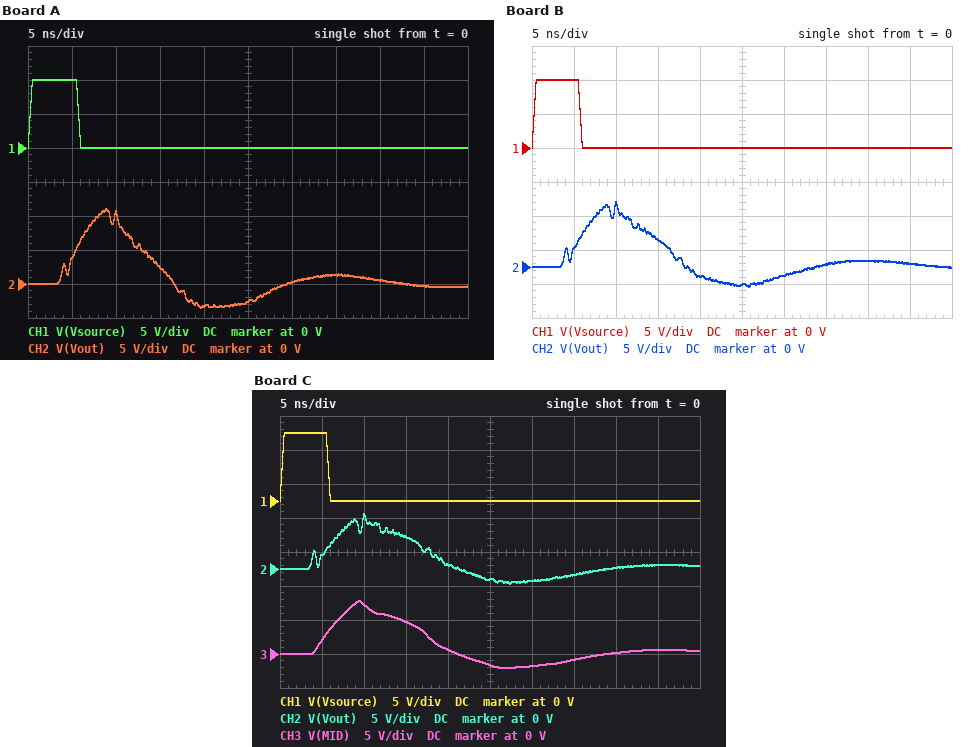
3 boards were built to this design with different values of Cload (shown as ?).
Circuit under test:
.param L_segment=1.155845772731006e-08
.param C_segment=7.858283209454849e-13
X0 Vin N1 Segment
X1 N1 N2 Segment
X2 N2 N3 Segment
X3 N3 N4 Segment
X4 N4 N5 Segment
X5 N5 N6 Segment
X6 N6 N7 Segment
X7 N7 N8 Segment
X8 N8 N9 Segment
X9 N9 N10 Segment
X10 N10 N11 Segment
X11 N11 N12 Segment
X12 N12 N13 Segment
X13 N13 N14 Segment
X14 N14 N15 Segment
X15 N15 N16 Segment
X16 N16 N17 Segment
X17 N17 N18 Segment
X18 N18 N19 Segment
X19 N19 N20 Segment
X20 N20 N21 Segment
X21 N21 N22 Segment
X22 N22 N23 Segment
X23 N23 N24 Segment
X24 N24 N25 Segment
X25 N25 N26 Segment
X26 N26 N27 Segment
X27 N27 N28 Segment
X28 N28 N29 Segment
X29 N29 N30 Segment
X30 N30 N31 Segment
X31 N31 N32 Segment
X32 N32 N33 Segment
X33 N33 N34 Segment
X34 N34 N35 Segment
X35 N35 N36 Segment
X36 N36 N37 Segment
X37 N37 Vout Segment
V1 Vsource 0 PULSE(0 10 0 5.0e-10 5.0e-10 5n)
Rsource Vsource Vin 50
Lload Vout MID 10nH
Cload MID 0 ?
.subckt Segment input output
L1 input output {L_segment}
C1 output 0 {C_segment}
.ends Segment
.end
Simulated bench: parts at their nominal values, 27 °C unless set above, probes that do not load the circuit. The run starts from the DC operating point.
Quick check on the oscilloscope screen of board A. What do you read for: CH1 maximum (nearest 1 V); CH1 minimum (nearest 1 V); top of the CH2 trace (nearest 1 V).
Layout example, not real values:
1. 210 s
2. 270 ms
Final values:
1. 10 V
2. 0 V
3. 11 V
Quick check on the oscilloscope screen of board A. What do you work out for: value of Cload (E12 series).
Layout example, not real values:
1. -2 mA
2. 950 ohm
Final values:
1. 27 pF
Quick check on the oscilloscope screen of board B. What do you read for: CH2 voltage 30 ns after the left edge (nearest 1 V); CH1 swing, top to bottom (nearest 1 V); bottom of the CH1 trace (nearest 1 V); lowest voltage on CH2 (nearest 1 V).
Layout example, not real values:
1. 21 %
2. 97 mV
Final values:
1. -1 V
2. 10 V
3. 0 V
4. -3 V
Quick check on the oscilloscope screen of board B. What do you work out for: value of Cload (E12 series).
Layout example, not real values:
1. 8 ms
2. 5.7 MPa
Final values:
1. 39 pF
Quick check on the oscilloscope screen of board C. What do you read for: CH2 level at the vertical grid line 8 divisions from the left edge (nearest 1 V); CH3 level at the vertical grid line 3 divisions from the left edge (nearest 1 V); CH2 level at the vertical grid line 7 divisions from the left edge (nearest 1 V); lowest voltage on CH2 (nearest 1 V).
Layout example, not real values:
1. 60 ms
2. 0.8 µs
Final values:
1. 0 V
2. 5 V
3. -1 V
4. -2 V
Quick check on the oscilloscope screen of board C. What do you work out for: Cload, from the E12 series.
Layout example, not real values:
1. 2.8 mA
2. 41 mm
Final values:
1. 56 pF
